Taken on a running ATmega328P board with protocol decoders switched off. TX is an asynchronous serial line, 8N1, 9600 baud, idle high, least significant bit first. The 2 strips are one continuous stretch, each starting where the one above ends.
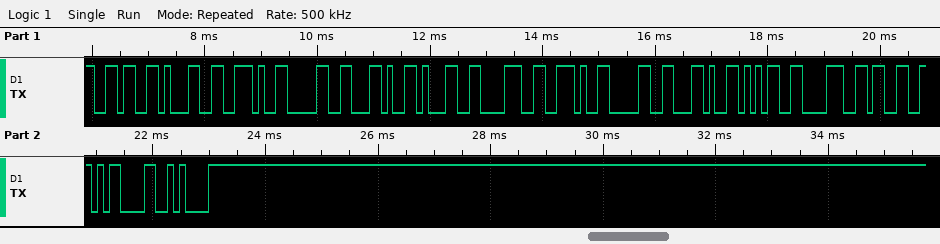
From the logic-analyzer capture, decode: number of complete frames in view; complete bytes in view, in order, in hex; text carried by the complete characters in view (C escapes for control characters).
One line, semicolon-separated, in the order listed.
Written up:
15; 36 31 2E 30 2C 31 38 2E 30 2C 35 38 33 0D 0A; "61.0,18.0,583\r\n"
